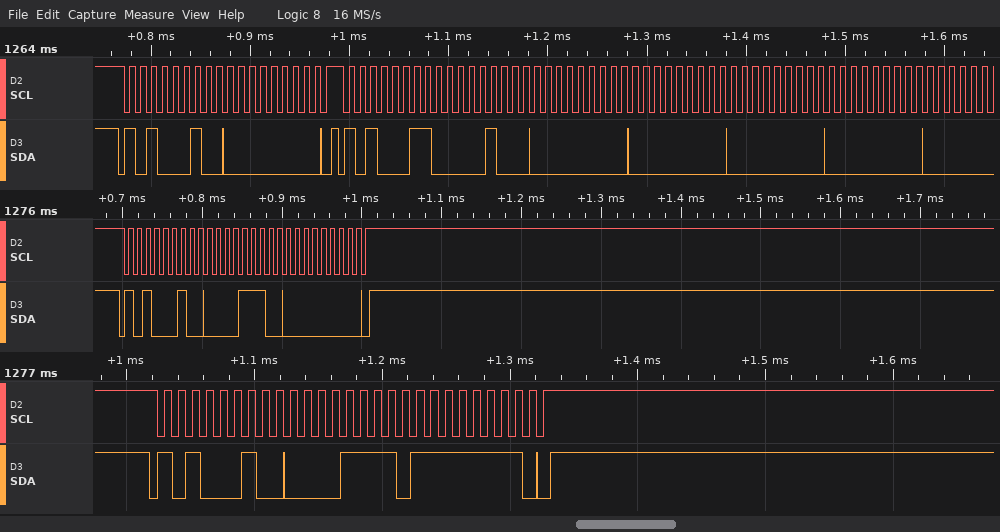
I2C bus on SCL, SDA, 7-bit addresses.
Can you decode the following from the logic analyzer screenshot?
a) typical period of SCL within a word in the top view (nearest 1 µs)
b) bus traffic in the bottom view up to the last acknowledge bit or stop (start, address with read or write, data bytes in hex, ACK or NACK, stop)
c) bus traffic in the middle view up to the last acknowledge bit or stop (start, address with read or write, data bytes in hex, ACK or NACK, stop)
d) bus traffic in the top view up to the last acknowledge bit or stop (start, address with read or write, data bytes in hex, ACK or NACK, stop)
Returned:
11 µs
start, address 51 write ACK, 0F ACK, FF ACK, stop
start, address 51 write ACK, 0E ACK, 00 ACK, stop
start, address 51 write ACK, 00 ACK, stop, start, address 51 read ACK, 08 ACK, 00 ACK, 00 ACK, 00 ACK, 00 ACK
